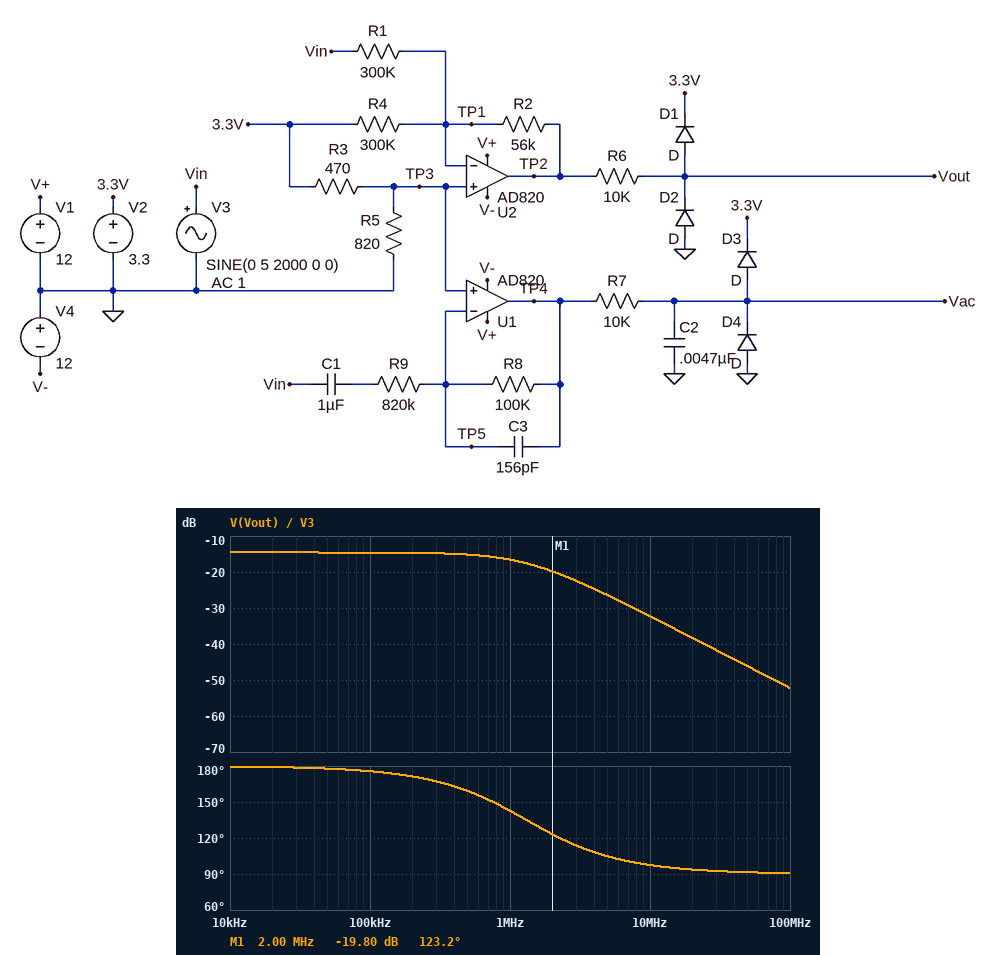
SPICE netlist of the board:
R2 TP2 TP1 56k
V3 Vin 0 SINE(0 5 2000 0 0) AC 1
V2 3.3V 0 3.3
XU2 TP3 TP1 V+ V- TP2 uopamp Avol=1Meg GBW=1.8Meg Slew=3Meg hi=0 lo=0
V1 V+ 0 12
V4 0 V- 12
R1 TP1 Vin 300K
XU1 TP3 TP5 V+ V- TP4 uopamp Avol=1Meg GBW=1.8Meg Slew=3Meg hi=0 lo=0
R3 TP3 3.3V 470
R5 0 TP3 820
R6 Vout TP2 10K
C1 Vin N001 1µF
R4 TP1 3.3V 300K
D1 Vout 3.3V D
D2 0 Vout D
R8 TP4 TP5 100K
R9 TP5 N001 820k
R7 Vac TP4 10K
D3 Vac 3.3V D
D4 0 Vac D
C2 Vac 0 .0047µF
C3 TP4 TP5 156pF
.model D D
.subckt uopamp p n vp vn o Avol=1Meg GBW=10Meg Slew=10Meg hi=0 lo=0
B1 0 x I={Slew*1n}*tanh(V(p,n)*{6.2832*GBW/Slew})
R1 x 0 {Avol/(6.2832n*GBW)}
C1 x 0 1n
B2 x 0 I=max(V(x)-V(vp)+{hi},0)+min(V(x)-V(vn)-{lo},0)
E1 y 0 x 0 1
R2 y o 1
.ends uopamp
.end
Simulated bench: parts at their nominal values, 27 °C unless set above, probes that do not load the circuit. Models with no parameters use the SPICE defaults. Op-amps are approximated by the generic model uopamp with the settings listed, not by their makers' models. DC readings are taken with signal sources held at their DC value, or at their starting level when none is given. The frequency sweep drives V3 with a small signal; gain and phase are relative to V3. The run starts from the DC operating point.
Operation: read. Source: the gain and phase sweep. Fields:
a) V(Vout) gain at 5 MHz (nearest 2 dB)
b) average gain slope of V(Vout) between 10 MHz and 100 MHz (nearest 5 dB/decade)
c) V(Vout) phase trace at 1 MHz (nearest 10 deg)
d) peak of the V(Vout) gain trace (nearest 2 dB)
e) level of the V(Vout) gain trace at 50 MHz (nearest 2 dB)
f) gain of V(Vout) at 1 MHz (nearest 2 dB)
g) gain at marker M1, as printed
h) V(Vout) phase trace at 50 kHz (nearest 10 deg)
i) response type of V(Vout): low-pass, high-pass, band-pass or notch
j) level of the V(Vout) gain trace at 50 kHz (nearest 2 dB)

-26 dB
-20 dB/decade
140 deg
-14 dB
-46 dB
-16 dB
-19.80 dB
180 deg
low-pass
-14 dB
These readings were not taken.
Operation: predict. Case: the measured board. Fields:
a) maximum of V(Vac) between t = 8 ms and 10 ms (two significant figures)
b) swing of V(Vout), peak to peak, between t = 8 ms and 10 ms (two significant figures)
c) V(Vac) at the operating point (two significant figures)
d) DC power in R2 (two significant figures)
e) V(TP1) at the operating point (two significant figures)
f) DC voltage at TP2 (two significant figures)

2.6 V
1.9 V
2.1 V
500 nW
2.1 V
2.3 V
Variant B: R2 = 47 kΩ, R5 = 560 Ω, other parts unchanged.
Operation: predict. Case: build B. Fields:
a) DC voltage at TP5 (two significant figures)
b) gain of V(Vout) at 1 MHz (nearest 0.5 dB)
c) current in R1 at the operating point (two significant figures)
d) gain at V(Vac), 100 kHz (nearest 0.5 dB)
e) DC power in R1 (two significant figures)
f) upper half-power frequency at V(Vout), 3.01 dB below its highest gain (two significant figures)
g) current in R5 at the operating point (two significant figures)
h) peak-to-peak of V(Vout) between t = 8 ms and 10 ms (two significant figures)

1.8 V
-18.0 dB
6.0 µA
-67.5 dB
11 µW
1.4 MHz
3.2 mA
1.6 V
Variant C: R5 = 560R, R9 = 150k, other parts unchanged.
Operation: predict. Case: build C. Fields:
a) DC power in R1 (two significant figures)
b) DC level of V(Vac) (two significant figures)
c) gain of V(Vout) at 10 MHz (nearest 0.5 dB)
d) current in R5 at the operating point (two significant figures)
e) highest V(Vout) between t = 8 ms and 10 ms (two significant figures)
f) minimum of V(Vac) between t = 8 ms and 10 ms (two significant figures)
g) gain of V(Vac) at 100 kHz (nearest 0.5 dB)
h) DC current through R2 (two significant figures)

11 µW
1.8 V
-32.5 dB
3.2 mA
2.8 V
-590 mV
-53.0 dB
960 nA
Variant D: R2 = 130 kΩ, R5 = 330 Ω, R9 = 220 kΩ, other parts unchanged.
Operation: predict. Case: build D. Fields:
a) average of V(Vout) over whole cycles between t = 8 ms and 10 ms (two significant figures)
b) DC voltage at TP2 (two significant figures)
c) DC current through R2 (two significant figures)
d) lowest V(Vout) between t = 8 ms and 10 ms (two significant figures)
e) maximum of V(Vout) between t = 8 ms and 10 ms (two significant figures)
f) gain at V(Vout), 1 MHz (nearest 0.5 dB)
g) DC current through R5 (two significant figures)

1.2 V
1.1 V
1.9 µA
-580 mV
3.3 V
-10.5 dB
4.1 mA
